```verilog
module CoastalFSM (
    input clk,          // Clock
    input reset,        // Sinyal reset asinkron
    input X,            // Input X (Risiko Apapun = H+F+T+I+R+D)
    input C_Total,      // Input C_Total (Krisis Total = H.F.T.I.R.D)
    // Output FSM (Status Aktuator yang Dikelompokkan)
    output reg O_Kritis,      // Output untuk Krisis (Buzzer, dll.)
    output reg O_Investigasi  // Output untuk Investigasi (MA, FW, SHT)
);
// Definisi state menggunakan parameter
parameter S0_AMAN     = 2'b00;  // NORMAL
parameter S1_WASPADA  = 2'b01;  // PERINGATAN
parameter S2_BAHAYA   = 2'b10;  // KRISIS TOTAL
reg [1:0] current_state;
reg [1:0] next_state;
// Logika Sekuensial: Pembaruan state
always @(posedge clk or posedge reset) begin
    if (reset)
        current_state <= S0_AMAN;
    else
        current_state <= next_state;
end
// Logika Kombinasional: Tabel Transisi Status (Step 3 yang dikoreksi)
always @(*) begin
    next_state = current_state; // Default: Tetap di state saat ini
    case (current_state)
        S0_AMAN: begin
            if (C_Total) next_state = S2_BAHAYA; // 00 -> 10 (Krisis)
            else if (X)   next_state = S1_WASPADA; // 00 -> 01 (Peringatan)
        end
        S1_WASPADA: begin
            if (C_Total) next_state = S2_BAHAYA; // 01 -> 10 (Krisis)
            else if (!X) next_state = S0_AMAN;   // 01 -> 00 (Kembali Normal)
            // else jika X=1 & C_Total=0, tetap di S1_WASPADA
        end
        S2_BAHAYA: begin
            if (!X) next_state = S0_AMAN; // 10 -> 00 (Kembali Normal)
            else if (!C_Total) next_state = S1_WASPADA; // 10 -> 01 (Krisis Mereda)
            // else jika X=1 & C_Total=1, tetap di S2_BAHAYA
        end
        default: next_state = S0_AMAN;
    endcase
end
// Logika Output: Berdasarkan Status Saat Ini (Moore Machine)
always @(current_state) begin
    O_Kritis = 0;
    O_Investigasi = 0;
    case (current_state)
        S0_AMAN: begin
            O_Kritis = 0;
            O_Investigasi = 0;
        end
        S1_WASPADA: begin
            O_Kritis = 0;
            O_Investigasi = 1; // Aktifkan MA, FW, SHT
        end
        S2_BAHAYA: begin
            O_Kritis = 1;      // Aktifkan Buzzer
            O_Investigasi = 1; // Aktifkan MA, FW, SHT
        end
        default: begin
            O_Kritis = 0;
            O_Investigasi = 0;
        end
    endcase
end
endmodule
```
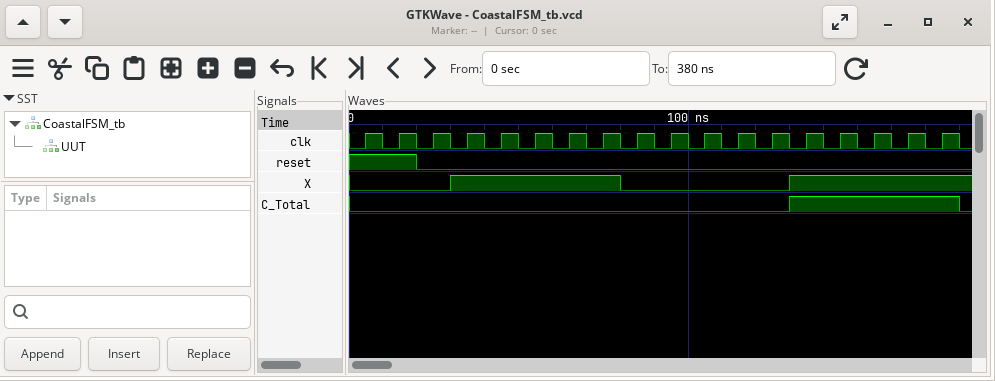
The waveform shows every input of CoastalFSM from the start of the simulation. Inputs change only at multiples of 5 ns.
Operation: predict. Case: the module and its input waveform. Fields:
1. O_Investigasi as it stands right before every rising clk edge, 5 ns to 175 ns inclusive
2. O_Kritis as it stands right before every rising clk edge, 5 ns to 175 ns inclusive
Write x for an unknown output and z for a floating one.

0 0 0 0 1 1 1 1 1 0 0 0 0 0 1 1 1 1
0 0 0 0 0 0 0 0 0 0 0 0 0 0 1 1 1 1
